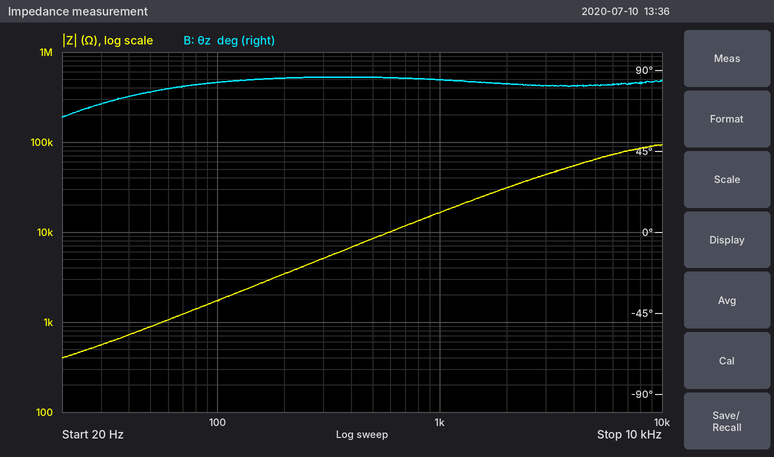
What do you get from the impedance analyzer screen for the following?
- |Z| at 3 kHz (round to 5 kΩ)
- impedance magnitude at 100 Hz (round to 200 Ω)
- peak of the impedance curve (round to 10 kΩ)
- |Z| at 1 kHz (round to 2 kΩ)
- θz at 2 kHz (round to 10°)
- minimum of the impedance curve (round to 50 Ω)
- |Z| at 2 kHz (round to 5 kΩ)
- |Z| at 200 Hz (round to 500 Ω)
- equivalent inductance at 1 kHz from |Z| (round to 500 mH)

45 kΩ
1.8 kΩ
90 kΩ
16 kΩ
80°
400 Ω
30 kΩ
3.5 kΩ
2.5 H
